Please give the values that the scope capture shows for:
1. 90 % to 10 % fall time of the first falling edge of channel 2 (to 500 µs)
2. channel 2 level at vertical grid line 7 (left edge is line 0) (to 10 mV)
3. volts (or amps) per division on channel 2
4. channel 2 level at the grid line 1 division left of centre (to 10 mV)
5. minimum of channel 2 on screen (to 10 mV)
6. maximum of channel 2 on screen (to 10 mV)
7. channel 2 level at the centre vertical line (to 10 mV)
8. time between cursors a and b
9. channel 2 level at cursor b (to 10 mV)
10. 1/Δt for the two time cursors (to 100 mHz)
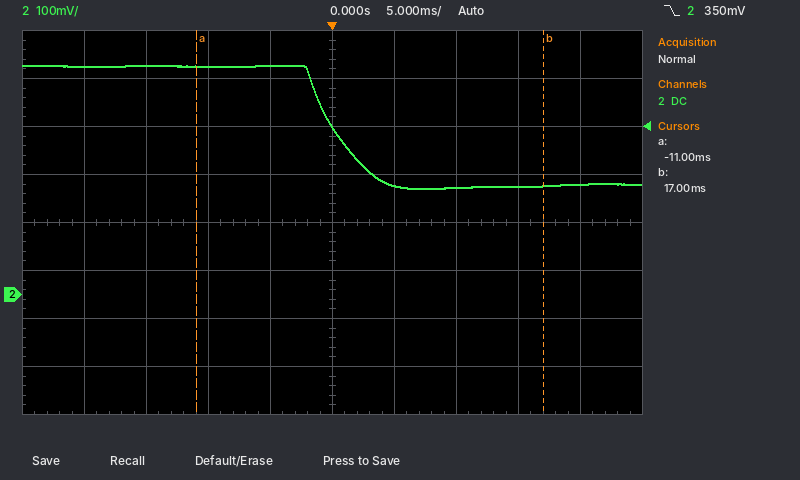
5.0 ms
220 mV
100 mV
480 mV
220 mV
480 mV
350 mV
28.0 ms
230 mV
35.7 Hz
